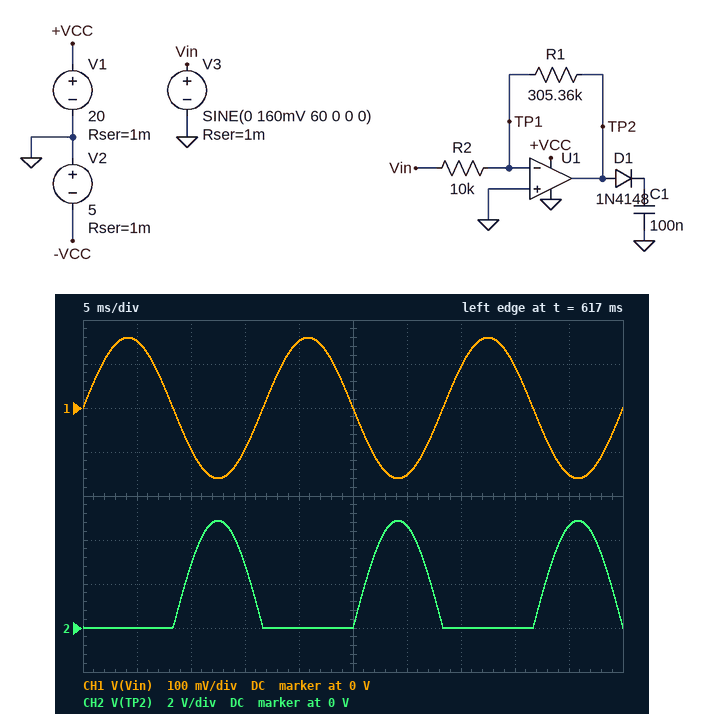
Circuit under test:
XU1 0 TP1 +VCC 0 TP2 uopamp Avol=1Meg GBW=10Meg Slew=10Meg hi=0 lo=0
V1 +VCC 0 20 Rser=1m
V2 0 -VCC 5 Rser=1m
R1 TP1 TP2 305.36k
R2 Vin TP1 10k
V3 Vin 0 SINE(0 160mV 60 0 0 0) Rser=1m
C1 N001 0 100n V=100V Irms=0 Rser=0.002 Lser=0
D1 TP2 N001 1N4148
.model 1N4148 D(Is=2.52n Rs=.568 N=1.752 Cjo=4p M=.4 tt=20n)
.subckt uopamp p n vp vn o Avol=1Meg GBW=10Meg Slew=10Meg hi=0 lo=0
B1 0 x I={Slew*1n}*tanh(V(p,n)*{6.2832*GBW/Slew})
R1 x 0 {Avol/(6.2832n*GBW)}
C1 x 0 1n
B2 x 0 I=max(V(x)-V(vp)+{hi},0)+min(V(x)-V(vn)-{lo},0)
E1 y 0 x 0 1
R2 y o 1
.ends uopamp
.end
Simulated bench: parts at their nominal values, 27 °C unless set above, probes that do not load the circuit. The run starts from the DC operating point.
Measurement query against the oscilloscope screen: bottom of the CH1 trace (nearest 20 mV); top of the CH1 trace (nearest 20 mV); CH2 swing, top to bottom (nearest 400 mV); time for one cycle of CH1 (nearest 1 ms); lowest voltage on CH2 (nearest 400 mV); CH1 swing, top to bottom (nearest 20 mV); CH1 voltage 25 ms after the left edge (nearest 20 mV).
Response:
-160 mV
160 mV
4.8 V
17 ms
0 V
320 mV
0 V
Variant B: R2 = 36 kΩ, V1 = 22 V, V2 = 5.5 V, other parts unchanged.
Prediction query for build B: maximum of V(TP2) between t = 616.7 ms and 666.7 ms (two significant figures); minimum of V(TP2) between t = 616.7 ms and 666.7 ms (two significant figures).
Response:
1.4 V
-7.1 mV
